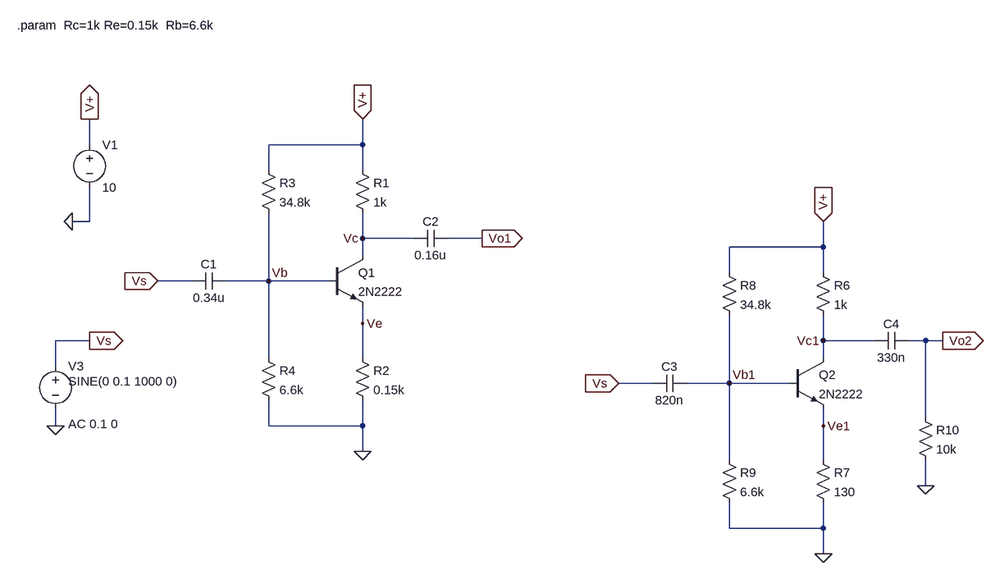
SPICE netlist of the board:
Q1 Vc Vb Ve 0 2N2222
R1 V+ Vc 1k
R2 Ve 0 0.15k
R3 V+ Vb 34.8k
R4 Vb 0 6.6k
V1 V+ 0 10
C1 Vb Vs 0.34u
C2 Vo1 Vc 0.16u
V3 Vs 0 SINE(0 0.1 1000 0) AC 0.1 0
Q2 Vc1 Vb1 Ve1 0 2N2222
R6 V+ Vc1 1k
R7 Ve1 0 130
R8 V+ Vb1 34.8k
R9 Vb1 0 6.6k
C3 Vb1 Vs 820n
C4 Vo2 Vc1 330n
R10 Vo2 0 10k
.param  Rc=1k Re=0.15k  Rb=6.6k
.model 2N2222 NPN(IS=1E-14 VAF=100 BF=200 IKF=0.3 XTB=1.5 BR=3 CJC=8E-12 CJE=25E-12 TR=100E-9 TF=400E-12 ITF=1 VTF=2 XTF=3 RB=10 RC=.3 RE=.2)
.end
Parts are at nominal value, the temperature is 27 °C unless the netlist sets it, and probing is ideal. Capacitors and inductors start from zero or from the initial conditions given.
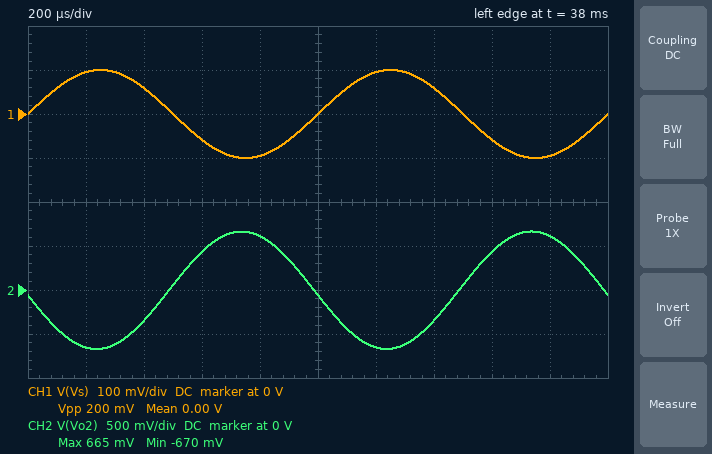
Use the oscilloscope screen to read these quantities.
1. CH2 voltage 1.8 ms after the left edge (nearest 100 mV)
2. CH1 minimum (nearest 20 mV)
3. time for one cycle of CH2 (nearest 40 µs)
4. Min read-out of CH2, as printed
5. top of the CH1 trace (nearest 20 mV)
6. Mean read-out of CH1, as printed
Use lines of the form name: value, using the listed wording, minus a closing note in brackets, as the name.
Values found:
CH2 voltage 1.8 ms after the left edge: 600 mV
CH1 minimum: -100 mV
time for one cycle of CH2: 1.00 ms
Min read-out of CH2, as printed: -670 mV
top of the CH1 trace: 100 mV
Mean read-out of CH1, as printed: 0.00 V
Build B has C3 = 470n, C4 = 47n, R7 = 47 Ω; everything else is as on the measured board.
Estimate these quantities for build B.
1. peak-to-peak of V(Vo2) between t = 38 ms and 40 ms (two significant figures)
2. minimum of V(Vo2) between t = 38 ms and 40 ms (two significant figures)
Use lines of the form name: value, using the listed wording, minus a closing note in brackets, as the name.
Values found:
peak-to-peak of V(Vo2) between t = 38 ms and 40 ms: 2.8 V
minimum of V(Vo2) between t = 38 ms and 40 ms: -1.4 V
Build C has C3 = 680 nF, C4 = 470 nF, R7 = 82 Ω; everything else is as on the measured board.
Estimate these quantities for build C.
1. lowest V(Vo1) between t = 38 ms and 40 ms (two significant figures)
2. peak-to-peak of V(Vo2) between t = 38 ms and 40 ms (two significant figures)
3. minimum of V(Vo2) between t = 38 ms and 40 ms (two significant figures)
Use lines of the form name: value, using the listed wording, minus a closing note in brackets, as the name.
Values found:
lowest V(Vo1) between t = 38 ms and 40 ms: 4.3 V
peak-to-peak of V(Vo2) between t = 38 ms and 40 ms: 2.1 V
minimum of V(Vo2) between t = 38 ms and 40 ms: -1.1 V
